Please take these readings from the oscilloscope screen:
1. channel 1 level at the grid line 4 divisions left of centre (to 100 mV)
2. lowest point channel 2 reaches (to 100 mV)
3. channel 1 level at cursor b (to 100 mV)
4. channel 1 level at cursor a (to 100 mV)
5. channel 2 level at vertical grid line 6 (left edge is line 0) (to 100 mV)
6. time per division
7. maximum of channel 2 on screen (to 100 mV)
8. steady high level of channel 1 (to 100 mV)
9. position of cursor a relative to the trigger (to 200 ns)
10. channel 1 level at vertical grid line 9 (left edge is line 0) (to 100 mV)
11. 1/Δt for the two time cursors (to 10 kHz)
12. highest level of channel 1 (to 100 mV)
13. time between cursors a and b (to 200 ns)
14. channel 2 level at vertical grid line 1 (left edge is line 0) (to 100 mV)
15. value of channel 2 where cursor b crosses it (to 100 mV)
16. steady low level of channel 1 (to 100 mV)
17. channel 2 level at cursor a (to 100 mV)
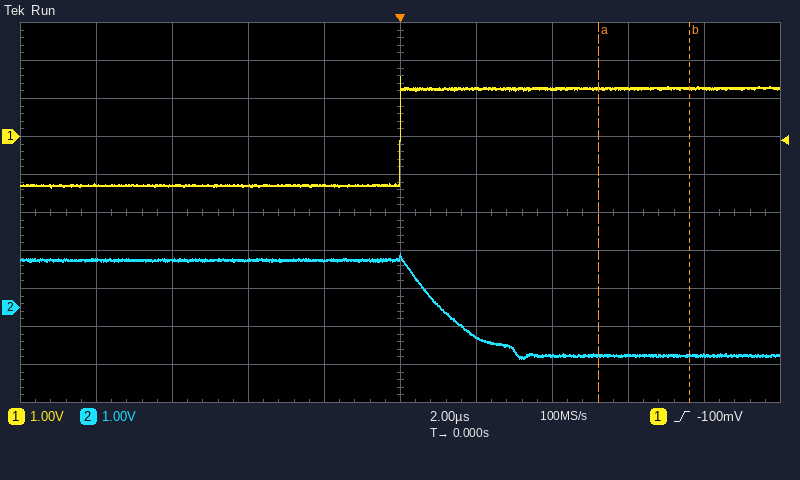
-1.3 V
-1.3 V
1.3 V
1.3 V
-800 mV
2 µs
1.4 V
1.3 V
+5.2 µs
1.3 V
420 kHz
1.6 V
2.4 µs
1.3 V
-1.3 V
-1.3 V
-1.3 V
